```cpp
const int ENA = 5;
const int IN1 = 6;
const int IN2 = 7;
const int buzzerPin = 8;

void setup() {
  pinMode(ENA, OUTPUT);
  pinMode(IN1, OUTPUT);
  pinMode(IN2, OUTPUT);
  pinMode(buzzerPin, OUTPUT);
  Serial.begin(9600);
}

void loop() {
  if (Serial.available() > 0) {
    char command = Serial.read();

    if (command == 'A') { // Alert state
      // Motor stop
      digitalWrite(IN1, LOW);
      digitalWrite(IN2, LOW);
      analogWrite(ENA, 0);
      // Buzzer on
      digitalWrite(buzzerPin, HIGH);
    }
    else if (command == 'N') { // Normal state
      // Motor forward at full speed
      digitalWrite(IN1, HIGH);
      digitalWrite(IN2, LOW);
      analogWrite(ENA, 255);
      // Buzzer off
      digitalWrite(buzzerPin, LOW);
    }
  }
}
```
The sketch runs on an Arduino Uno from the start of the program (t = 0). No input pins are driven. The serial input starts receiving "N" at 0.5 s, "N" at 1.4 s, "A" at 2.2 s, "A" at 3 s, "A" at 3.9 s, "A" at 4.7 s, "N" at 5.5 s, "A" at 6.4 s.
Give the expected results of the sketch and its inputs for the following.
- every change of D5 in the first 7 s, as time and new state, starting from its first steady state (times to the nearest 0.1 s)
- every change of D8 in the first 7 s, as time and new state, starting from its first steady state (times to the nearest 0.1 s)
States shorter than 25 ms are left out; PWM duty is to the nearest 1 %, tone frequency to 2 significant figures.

0 s low; 0.5 s high; 2.2 s low; 5.5 s high; 6.4 s low
0 s low; 2.2 s high; 5.5 s low; 6.4 s high
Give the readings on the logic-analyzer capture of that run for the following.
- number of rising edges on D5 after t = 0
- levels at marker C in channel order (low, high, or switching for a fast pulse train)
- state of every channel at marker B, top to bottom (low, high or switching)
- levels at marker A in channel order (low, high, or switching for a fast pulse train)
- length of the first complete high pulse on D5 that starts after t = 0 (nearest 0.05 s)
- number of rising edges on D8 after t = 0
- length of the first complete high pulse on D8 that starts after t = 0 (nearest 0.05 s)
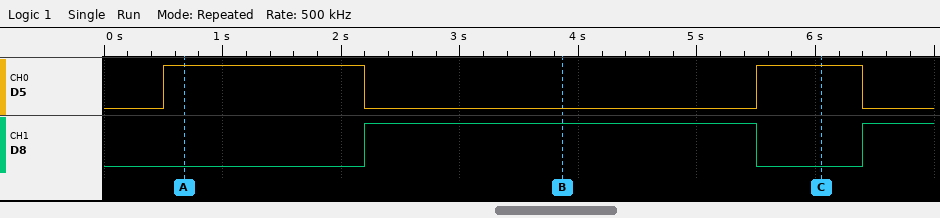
2
D5 high, D8 low
D5 low, D8 high
D5 high, D8 low
1.70 s
2
3.30 s
